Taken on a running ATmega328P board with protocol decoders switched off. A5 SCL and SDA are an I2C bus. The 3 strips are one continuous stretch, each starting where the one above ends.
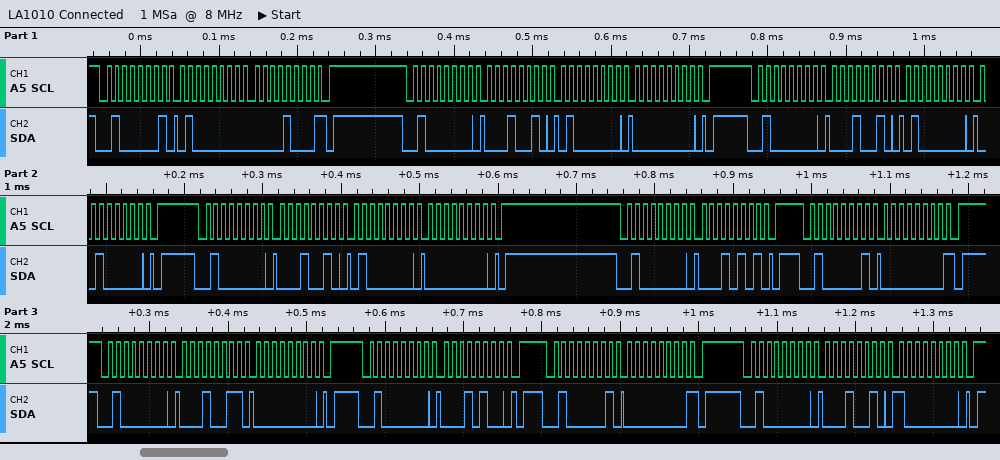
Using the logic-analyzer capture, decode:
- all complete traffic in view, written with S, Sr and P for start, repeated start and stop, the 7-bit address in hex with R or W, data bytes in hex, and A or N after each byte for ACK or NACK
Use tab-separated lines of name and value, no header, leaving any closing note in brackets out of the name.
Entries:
all complete traffic in view, written with S, Sr and P for start, repeated start and stop, the 7-bit address in hex with R or W, data bytes in hex, and A or N after each byte for ACK or NACK	S 20R A 40 A 08 N P S 20W A 12 A 40 A 00 A P S 20W A 12 A 40 A 20 A P S 20W A 12 A 40 A 00 A P S 20W A 15 A P S 20R A 00 N P S 20W A 13 A 00 A P S 20W A 14 A P S 20R A 00 N P S 20W A 12 A 80 A P
